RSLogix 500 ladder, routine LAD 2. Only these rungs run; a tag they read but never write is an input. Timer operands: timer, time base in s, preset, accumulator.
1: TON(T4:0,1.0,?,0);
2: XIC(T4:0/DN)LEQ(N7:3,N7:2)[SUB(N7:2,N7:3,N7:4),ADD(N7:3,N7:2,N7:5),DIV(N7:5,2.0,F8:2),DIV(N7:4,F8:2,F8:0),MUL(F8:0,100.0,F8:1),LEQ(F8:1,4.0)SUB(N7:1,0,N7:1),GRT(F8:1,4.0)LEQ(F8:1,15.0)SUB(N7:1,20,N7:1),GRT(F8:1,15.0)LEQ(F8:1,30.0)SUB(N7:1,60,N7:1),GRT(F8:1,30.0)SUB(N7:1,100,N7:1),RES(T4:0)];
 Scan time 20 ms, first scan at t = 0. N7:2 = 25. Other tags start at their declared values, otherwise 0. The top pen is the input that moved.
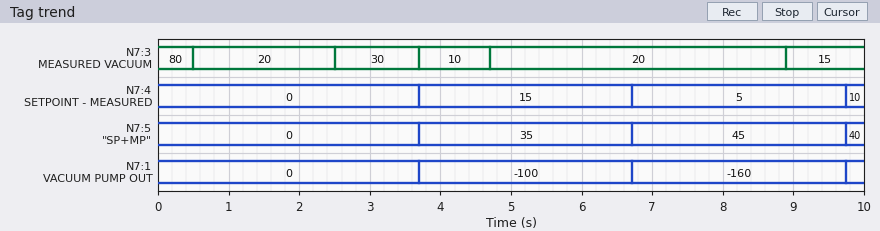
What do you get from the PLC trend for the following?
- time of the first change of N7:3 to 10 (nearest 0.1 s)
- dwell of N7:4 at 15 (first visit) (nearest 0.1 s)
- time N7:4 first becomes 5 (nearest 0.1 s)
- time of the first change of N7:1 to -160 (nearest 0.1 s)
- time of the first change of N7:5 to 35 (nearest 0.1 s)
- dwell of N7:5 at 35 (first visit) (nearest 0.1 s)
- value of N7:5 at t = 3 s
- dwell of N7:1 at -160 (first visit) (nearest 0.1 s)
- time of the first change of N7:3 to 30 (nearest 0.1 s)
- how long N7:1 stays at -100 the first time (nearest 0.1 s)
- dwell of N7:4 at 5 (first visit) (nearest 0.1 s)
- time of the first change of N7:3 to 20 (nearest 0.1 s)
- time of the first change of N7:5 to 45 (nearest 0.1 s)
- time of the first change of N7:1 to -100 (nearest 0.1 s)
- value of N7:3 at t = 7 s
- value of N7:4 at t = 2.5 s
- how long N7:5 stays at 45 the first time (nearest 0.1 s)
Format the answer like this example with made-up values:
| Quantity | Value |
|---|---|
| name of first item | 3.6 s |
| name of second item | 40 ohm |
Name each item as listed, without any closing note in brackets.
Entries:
| Quantity | Value |
|---|---|
| time of the first change of N7:3 to 10 | 3.7 s |
| dwell of N7:4 at 15 (first visit) | 3.0 s |
| time N7:4 first becomes 5 | 6.7 s |
| time of the first change of N7:1 to -160 | 6.7 s |
| time of the first change of N7:5 to 35 | 3.7 s |
| dwell of N7:5 at 35 (first visit) | 3.0 s |
| value of N7:5 at t = 3 s | 0 |
| dwell of N7:1 at -160 (first visit) | 3.0 s |
| time of the first change of N7:3 to 30 | 2.5 s |
| how long N7:1 stays at -100 the first time | 3.0 s |
| dwell of N7:4 at 5 (first visit) | 3.0 s |
| time of the first change of N7:3 to 20 | 0.5 s |
| time of the first change of N7:5 to 45 | 6.7 s |
| time of the first change of N7:1 to -100 | 3.7 s |
| value of N7:3 at t = 7 s | 20 |
| value of N7:4 at t = 2.5 s | 0 |
| how long N7:5 stays at 45 the first time | 3.0 s |
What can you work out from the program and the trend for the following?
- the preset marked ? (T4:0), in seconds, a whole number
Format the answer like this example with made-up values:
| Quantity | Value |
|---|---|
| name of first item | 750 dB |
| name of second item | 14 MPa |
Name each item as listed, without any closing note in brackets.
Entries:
| Quantity | Value |
|---|---|
| the preset marked ? (T4:0), in seconds, a whole number | 3 s |
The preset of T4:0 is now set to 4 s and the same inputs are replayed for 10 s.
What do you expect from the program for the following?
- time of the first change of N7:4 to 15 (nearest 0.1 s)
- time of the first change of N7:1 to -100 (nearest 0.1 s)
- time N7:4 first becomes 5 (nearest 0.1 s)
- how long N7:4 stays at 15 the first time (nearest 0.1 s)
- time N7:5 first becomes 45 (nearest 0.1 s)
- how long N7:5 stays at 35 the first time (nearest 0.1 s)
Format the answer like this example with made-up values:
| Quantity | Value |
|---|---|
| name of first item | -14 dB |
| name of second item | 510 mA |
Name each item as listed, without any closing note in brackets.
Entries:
| Quantity | Value |
|---|---|
| time of the first change of N7:4 to 15 | 4.0 s |
| time of the first change of N7:1 to -100 | 4.0 s |
| time N7:4 first becomes 5 | 8.0 s |
| how long N7:4 stays at 15 the first time | 4.0 s |
| time N7:5 first becomes 45 | 8.0 s |
| how long N7:5 stays at 35 the first time | 4.0 s |
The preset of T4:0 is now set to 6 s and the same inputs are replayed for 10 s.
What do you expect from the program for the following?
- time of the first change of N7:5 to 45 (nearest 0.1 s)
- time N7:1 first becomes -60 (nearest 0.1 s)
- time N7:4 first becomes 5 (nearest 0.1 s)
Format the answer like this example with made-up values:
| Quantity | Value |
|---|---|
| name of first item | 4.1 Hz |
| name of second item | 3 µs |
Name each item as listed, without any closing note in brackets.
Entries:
| Quantity | Value |
|---|---|
| time of the first change of N7:5 to 45 | 6.0 s |
| time N7:1 first becomes -60 | 6.0 s |
| time N7:4 first becomes 5 | 6.0 s |
